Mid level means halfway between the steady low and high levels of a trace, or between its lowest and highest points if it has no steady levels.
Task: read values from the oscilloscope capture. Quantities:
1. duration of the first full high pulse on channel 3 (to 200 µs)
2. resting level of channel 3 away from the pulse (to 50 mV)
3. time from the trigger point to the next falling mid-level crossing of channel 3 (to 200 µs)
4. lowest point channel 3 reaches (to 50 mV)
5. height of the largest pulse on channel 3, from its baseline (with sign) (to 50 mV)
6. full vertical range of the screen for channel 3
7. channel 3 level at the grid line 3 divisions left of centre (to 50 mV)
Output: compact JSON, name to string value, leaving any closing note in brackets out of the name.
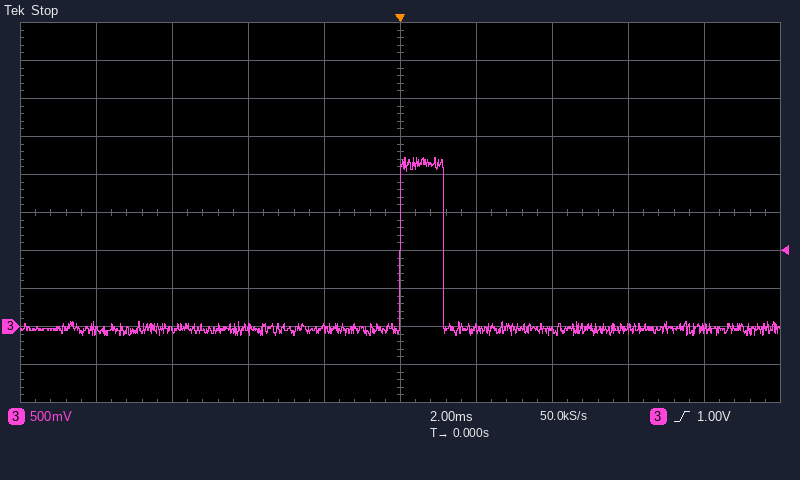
{"duration of the first full high pulse on channel 3": "1.2 ms", "resting level of channel 3 away from the pulse": "-50 mV", "time from the trigger point to the next falling mid-level crossing of channel 3": "1.2 ms", "lowest point channel 3 reaches": "-100 mV", "height of the largest pulse on channel 3, from its baseline (with sign)": "+2.25 V", "full vertical range of the screen for channel 3": "5 V", "channel 3 level at the grid line 3 divisions left of centre": "-50 mV"}
